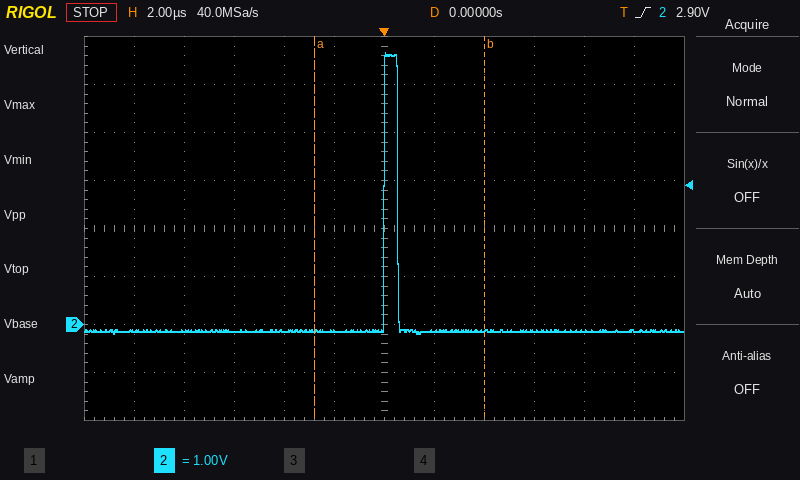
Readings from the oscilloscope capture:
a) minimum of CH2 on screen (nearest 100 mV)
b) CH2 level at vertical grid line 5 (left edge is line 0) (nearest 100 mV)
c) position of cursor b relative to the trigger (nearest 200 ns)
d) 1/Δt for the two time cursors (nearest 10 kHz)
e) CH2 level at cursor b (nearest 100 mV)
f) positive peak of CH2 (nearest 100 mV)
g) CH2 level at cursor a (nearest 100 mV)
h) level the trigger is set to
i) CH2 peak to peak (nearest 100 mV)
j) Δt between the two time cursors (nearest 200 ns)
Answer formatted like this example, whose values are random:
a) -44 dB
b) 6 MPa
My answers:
a) -200 mV
b) -100 mV
c) +4.0 µs
d) 150 kHz
e) -100 mV
f) 5.7 V
g) -100 mV
h) 2.90 V
i) 5.9 V
j) 6.8 µs
